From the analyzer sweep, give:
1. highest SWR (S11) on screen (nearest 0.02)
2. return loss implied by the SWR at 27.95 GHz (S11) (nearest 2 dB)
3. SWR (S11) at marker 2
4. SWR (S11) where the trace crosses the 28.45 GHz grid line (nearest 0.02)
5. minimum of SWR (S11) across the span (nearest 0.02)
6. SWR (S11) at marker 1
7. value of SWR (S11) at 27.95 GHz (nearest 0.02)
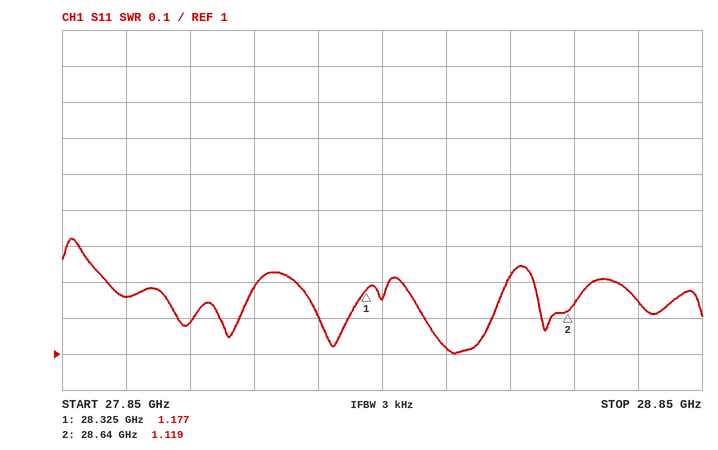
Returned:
1.32
22 dB
1.119
1.02
1.00
1.177
1.16
